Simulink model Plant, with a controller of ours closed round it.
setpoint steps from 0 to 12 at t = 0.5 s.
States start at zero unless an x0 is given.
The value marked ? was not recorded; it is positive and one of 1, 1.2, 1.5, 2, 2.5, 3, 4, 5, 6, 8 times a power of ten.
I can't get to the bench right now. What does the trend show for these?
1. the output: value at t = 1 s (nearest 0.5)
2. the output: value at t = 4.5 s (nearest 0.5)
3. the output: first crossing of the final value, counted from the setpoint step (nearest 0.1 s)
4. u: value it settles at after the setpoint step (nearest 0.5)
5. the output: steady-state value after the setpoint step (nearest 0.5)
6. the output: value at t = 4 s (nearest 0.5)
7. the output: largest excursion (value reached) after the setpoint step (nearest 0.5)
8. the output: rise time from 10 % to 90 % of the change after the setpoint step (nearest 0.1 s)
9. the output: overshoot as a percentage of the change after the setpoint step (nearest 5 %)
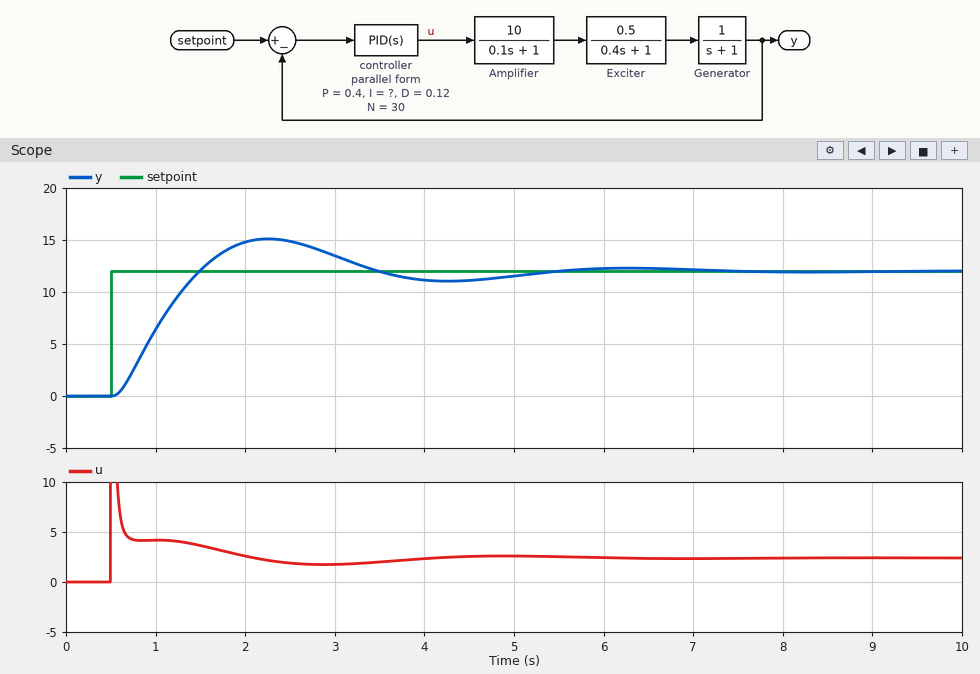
6.5
11.0
1.0 s
2.5
12.0
11.0
15.0
0.7 s
25 %
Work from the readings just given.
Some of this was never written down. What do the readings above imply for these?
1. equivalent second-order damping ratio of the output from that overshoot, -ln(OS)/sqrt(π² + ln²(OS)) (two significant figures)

0.40
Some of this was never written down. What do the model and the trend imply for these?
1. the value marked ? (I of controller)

0.8
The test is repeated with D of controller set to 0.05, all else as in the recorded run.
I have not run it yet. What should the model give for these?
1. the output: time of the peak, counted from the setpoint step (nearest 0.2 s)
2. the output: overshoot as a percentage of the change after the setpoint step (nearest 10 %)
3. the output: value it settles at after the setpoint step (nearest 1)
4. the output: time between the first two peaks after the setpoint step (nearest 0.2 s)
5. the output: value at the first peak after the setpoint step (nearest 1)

1.6 s
40 %
12
3.4 s
17
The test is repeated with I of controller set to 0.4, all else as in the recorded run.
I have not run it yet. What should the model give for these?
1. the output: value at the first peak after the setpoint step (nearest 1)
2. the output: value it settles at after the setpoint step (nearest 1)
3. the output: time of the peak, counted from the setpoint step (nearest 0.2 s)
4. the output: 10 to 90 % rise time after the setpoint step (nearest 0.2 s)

13
12
2.4 s
1.0 s
